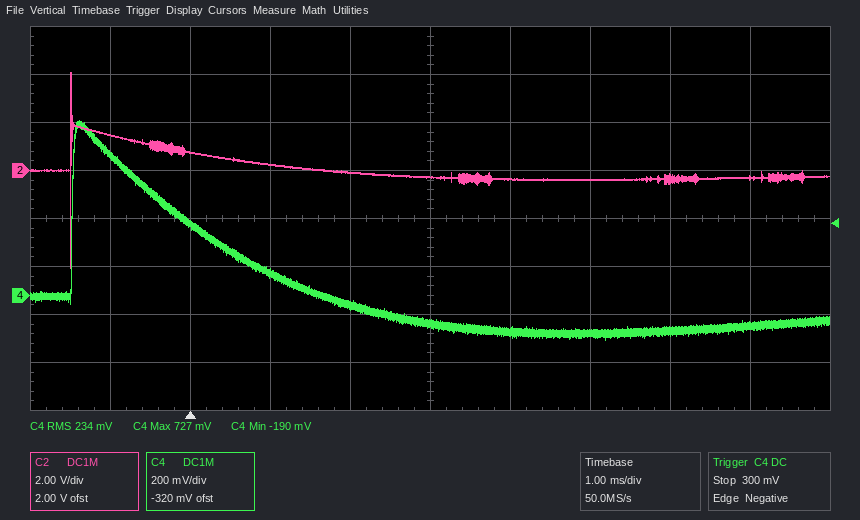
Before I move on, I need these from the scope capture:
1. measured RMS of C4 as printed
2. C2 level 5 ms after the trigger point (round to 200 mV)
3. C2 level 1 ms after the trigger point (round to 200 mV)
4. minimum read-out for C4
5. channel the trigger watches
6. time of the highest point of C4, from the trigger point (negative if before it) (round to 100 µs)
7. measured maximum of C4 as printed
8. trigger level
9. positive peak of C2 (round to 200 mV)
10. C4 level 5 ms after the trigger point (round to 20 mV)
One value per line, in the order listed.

234 mV
-400 mV
200 mV
-190 mV
C4
-1.4 ms
727 mV
300 mV
4.0 V
-160 mV
